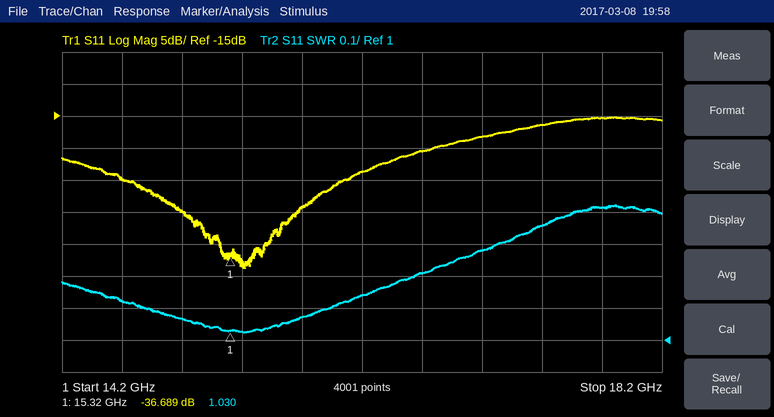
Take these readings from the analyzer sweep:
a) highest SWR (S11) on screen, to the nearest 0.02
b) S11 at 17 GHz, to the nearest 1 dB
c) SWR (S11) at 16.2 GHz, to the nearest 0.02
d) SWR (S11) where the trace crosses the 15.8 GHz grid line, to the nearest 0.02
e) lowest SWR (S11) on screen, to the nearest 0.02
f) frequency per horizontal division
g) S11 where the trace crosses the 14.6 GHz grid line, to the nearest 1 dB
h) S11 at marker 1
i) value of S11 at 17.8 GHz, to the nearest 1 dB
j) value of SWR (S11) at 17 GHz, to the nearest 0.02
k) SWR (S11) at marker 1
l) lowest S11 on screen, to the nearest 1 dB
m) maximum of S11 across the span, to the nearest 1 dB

1.42
-18 dB
1.14
1.08
1.02
400 MHz
-25 dB
-36.689 dB
-15 dB
1.28
1.030
-39 dB
-15 dB
